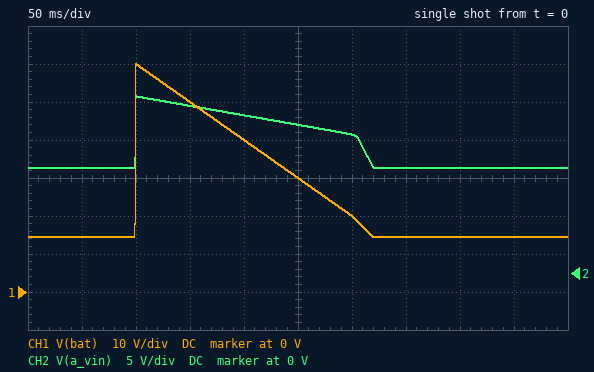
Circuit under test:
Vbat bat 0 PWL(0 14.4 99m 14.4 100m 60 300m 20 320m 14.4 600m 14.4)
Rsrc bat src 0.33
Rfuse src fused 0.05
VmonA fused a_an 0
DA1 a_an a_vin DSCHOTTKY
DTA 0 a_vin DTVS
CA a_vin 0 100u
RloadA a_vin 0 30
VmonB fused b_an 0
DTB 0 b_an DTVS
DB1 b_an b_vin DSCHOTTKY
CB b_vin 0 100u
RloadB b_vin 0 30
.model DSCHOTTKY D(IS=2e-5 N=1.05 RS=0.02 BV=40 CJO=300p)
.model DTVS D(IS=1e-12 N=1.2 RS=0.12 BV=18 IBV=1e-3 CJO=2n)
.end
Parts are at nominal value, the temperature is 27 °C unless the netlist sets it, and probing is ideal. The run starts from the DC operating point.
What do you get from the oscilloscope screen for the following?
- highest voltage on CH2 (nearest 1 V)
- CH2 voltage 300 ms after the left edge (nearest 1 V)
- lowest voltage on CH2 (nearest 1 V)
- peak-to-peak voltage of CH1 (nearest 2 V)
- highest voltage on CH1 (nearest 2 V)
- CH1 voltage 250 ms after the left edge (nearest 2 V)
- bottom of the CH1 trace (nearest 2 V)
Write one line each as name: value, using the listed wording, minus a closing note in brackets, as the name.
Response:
highest voltage on CH2: 23 V
CH2 voltage 300 ms after the left edge: 18 V
lowest voltage on CH2: 14 V
peak-to-peak voltage of CH1: 46 V
highest voltage on CH1: 60 V
CH1 voltage 250 ms after the left edge: 30 V
bottom of the CH1 trace: 14 V
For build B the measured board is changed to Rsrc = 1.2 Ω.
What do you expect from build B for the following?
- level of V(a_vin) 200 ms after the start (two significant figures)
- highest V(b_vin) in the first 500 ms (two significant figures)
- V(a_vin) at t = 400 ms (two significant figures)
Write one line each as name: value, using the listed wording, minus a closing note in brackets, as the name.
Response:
level of V(a_vin) 200 ms after the start: 19 V
highest V(b_vin) in the first 500 ms: 20 V
V(a_vin) at t = 400 ms: 13 V
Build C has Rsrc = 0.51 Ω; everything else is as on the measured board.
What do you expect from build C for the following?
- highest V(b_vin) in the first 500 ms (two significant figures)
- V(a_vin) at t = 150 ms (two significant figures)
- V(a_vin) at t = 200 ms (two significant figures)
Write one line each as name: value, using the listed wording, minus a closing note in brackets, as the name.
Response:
highest V(b_vin) in the first 500 ms: 22 V
V(a_vin) at t = 150 ms: 21 V
V(a_vin) at t = 200 ms: 20 V
